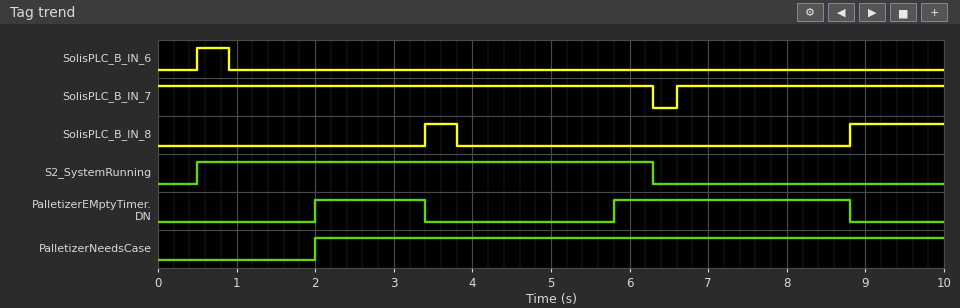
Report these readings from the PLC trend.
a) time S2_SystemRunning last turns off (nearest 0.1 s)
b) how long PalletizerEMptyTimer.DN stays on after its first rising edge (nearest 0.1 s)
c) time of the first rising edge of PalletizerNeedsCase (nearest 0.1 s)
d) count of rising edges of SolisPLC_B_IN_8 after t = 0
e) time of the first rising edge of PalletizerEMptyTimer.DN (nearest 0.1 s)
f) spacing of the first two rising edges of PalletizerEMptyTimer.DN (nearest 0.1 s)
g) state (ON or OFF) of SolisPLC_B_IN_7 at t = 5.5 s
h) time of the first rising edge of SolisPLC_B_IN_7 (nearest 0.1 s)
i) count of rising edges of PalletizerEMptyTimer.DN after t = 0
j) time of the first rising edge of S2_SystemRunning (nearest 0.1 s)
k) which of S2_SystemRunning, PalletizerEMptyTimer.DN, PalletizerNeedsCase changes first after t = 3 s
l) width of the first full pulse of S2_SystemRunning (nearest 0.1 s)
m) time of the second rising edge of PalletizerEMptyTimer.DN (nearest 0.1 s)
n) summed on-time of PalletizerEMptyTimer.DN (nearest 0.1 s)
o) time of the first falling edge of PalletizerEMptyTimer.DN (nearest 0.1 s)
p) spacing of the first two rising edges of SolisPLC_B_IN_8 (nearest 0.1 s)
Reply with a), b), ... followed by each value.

a) 6.3 s
b) 1.4 s
c) 2.0 s
d) 2
e) 2.0 s
f) 3.8 s
g) ON
h) 6.6 s
i) 2
j) 0.5 s
k) PalletizerEMptyTimer.DN
l) 5.8 s
m) 5.8 s
n) 4.4 s
o) 3.4 s
p) 5.4 s
